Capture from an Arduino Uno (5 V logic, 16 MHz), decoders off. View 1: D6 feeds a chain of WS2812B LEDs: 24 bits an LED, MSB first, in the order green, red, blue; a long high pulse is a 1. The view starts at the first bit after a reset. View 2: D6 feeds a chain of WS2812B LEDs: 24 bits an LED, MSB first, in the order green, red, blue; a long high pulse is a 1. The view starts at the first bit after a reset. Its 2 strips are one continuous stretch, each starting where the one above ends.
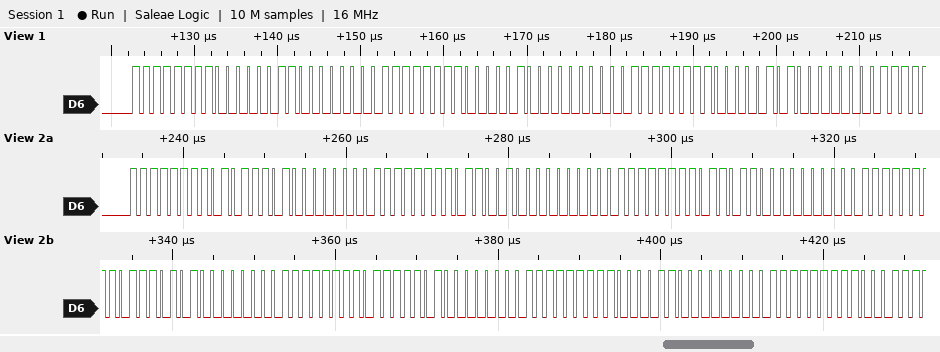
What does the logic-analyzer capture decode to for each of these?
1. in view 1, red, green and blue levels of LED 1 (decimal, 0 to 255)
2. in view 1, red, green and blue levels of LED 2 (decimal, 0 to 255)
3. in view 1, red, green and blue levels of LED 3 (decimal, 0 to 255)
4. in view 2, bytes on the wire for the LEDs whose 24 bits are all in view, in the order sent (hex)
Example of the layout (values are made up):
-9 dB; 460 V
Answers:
3, 255, 0; 4, 255, 0; 5, 255, 0; FF 5D 00 FF 64 00 FF 6C 00 FF 75 00 FF 7D 00 FF 86 00
